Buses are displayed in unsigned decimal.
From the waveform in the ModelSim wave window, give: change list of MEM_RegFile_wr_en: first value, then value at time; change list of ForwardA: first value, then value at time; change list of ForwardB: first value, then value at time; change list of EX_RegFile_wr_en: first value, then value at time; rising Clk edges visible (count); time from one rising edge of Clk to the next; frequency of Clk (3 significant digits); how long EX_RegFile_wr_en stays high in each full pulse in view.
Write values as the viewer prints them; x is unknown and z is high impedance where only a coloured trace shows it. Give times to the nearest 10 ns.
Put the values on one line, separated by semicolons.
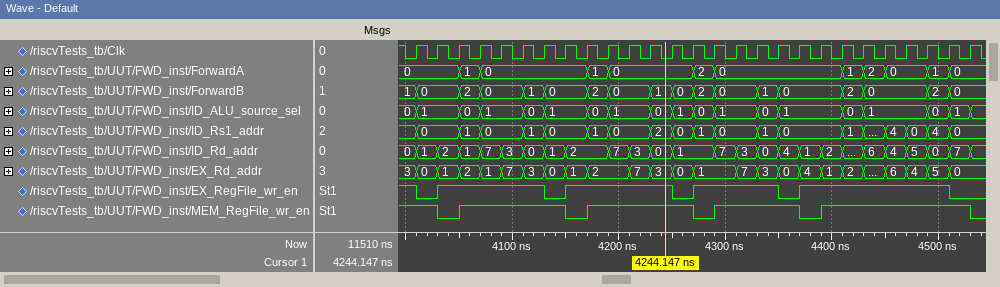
1, 0 at 4030 ns, 1 at 4050 ns, 0 at 4150 ns, 1 at 4170 ns, 0 at 4270 ns, 1 at 4290 ns, 0 at 4370 ns, 1 at 4390 ns, 0 at 4530 ns; 0, 1 at 4050 ns, 0 at 4070 ns, 1 at 4170 ns, 0 at 4190 ns, 2 at 4270 ns, 0 at 4290 ns, 1 at 4410 ns, 2 at 4430 ns, 0 at 4450 ns, 1 at 4490 ns, 0 at 4510 ns; 1, 0 at 4010 ns, 2 at 4050 ns, 0 at 4070 ns, 1 at 4110 ns, 0 at 4130 ns, 2 at 4170 ns, 0 at 4190 ns, 1 at 4230 ns, 0 at 4250 ns, 2 at 4270 ns, 0 at 4290 ns, 1 at 4330 ns, 0 at 4350 ns, 2 at 4410 ns, 0 at 4430 ns, 2 at 4490 ns, 0 at 4510 ns; 1, 0 at 4010 ns, 1 at 4030 ns, 0 at 4130 ns, 1 at 4150 ns, 0 at 4250 ns, 1 at 4270 ns, 0 at 4350 ns, 1 at 4370 ns, 0 at 4510 ns; 27; 20 ns; 50.0 MHz; 100 ns, 100 ns, 80 ns, 140 ns
